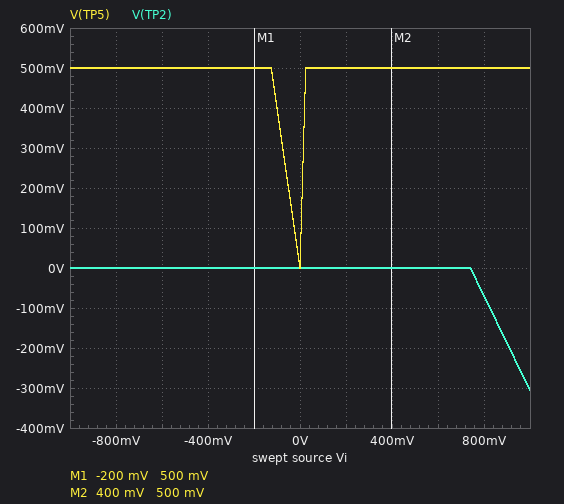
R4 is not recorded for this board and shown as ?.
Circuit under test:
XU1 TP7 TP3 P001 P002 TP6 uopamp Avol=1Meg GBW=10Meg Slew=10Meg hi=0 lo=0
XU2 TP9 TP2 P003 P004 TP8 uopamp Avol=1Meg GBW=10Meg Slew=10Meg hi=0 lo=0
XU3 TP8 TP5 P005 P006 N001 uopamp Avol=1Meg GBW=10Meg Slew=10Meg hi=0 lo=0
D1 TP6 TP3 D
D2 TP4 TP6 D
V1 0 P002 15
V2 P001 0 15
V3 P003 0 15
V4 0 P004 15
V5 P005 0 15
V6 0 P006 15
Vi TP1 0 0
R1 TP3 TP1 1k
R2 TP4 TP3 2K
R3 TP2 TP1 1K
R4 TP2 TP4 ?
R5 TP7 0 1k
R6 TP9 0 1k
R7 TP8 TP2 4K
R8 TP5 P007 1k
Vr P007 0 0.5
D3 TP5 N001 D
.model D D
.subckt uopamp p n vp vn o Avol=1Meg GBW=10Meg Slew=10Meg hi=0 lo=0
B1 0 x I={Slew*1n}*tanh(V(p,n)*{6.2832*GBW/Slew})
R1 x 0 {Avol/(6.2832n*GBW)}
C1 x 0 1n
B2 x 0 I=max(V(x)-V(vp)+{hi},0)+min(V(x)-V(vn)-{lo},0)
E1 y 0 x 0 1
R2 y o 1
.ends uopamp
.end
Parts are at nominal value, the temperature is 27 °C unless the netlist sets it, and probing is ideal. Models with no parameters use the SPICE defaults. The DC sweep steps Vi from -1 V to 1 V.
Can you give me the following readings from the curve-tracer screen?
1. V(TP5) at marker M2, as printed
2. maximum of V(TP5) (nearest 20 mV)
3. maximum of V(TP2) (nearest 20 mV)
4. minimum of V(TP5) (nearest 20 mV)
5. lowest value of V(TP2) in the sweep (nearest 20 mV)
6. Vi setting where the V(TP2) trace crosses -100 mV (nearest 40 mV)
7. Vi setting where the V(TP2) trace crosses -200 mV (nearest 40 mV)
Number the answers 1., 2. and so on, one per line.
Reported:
1. 500 mV
2. 500 mV
3. 0 V
4. 0 V
5. -300 mV
6. 840 mV
7. 920 mV
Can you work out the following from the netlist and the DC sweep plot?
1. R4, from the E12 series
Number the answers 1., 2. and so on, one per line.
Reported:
1. 330 Ω
